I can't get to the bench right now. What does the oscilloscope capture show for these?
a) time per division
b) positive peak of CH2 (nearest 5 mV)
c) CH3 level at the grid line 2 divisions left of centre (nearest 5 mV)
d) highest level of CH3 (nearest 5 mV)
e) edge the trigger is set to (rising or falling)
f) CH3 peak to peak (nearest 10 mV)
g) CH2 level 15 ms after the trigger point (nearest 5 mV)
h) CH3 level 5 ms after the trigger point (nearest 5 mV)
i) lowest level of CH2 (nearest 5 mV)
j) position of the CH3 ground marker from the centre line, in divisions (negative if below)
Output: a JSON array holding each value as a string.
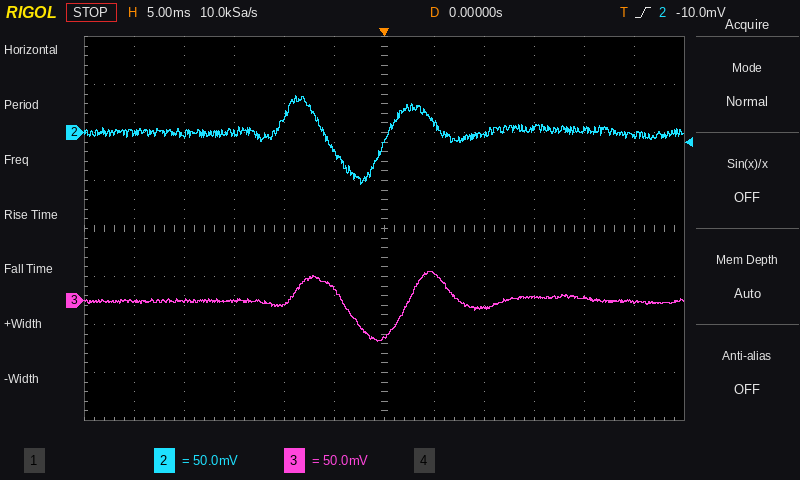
["5 ms", "40 mV", "-5 mV", "30 mV", "rising", "70 mV", "5 mV", "30 mV", "-55 mV", "-1.5 div"]
